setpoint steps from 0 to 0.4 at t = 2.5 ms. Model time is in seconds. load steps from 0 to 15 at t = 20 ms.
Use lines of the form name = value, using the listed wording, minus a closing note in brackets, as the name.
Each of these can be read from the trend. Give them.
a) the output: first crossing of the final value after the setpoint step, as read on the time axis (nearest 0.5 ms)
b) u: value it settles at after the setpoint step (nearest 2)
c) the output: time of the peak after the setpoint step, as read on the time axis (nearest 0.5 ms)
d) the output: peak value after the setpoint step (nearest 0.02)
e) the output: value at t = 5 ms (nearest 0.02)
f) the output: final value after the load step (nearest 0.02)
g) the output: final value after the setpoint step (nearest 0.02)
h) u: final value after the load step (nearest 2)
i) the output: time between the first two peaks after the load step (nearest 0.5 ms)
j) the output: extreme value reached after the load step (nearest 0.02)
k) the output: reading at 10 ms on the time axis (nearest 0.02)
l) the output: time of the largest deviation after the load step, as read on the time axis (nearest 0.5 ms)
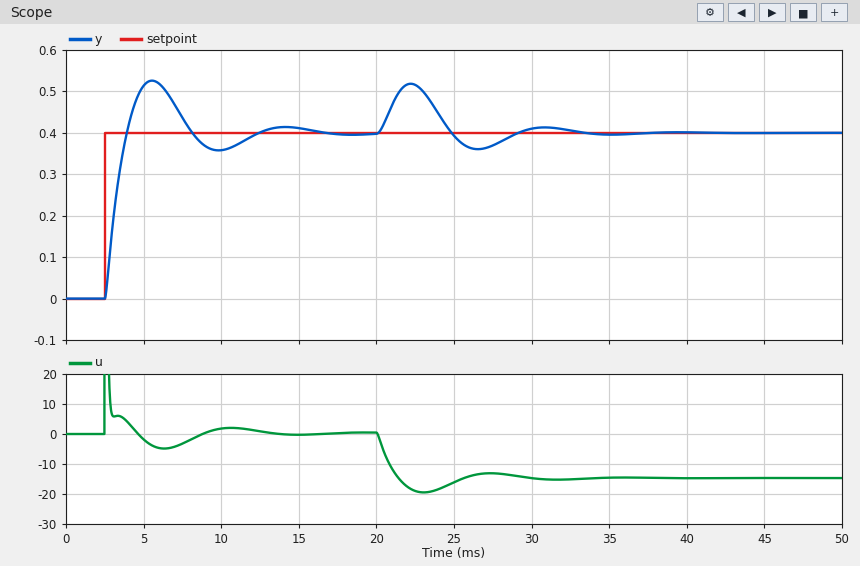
the output: first crossing of the final value after the setpoint step, as read on the time axis = 4.0 ms
u: value it settles at after the setpoint step = 0
the output: time of the peak after the setpoint step, as read on the time axis = 5.5 ms
the output: peak value after the setpoint step = 0.52
the output: value at t = 5 ms = 0.52
the output: final value after the load step = 0.40
the output: final value after the setpoint step = 0.40
u: final value after the load step = -14
the output: time between the first two peaks after the load step = 8.5 ms
the output: extreme value reached after the load step = 0.52
the output: reading at 10 ms on the time axis = 0.36
the output: time of the largest deviation after the load step, as read on the time axis = 22.0 ms
